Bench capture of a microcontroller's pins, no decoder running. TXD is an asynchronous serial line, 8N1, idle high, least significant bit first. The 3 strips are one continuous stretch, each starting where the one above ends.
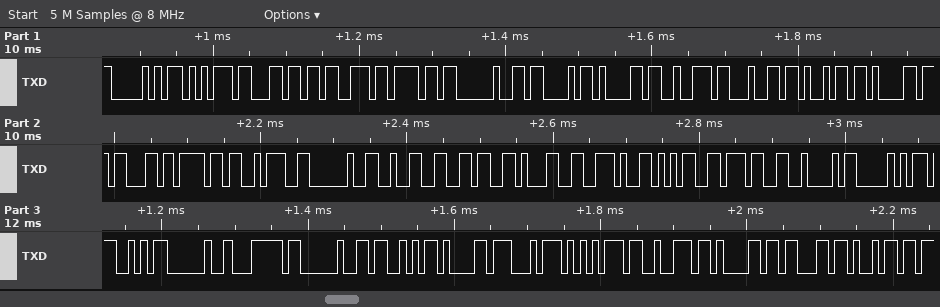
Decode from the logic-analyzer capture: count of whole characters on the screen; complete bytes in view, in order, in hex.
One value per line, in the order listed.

36
50 75 6C 73 6F 20 43 61 72 64 69 61 63 6F 3A 20 32 36 31 2E 35 37 42 50 53 20 7C 20 53 61 74 75 72 61 63 69
